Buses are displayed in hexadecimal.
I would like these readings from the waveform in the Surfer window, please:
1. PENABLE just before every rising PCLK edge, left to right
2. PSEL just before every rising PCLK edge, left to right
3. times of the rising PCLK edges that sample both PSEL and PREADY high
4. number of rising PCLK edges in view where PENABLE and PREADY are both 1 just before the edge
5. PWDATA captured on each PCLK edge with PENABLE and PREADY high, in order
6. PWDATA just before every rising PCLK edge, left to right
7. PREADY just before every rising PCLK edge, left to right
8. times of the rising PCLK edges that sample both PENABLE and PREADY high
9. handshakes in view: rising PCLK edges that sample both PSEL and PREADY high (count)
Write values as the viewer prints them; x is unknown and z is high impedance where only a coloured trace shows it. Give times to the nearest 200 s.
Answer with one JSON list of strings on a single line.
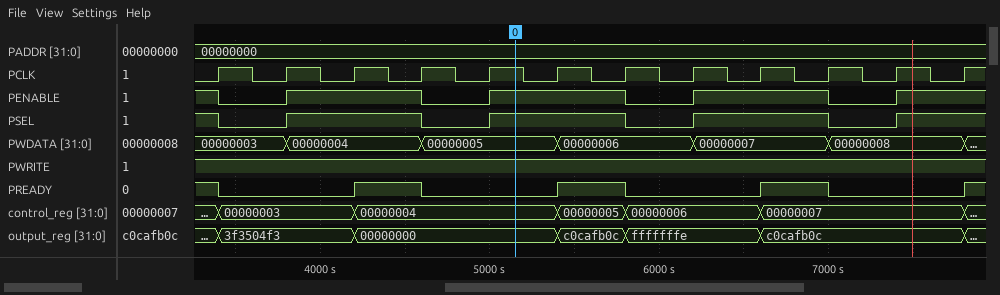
["1 0 1 1 0 1 1 0 1 1 0 1", "1 0 1 1 0 1 1 0 1 1 0 1", "3400 s, 4600 s, 5800 s, 7000 s", "4", "00000003, 00000004, 00000006, 00000007", "00000003, 00000003, 00000004, 00000004, 00000005, 00000005, 00000006, 00000006, 00000007, 00000007, 00000008, 00000008", "1 0 0 1 0 0 1 0 0 1 0 0", "3400 s, 4600 s, 5800 s, 7000 s", "4"]
